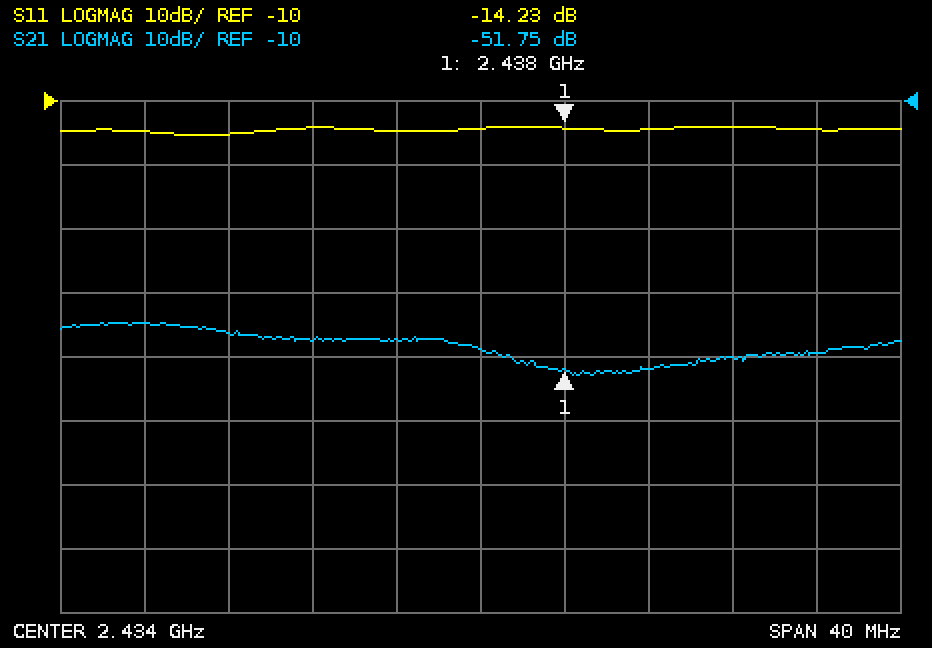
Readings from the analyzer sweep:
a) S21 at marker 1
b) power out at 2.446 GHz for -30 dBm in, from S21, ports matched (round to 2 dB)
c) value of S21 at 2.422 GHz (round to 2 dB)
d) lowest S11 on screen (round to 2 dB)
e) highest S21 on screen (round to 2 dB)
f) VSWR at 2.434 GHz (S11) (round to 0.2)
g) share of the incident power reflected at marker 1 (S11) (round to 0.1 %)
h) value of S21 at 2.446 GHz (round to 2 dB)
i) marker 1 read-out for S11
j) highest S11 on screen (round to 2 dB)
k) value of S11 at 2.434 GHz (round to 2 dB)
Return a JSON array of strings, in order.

["-51.75 dB", "-80 dBm", "-46 dB", "-16 dB", "-44 dB", "1.4", "3.8 %", "-50 dB", "-14.23 dB", "-14 dB", "-14 dB"]
